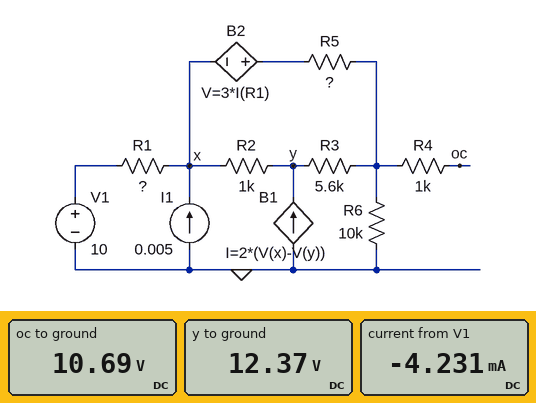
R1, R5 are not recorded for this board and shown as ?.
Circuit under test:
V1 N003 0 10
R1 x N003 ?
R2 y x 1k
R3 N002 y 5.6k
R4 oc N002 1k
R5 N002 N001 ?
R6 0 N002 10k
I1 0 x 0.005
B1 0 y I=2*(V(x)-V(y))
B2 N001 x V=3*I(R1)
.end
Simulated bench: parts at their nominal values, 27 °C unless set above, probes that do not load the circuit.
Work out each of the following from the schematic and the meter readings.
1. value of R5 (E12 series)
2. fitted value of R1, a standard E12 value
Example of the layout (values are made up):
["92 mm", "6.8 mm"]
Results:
["2.2 kΩ", "560 Ω"]
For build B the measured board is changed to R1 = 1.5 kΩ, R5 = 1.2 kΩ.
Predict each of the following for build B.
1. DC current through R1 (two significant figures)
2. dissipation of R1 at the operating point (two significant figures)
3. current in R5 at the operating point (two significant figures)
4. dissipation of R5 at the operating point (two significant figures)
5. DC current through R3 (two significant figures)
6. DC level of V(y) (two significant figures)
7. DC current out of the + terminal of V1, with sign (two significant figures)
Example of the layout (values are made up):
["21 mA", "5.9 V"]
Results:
["3.8 mA", "22 mW", "1.2 mA", "1.7 mW", "250 µA", "16 V", "-3.8 mA"]
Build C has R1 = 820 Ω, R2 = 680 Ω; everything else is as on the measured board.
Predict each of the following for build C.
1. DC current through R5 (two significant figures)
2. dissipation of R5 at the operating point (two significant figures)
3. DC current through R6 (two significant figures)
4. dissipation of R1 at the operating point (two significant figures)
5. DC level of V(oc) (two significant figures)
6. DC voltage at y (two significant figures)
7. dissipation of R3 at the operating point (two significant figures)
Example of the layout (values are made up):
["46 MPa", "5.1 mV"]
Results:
["830 µA", "1.5 mW", "1.2 mA", "14 mW", "12 V", "13 V", "590 µW"]
